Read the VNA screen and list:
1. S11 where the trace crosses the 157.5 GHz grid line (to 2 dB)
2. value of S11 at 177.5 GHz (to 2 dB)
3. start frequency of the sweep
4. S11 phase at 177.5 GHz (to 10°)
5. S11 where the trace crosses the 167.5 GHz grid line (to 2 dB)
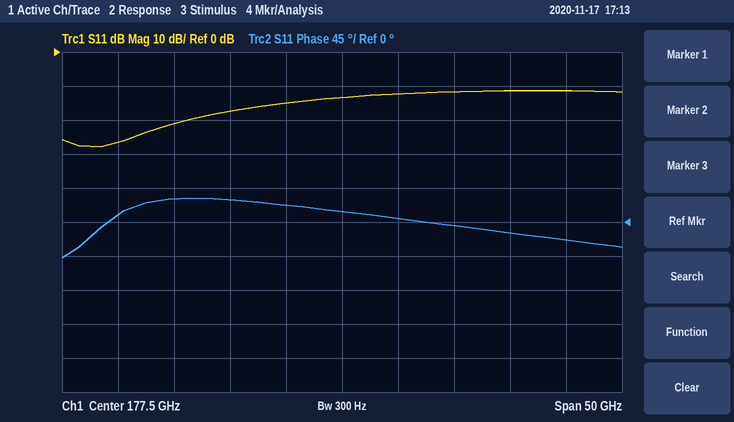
-26 dB
-14 dB
152.5 GHz
10°
-18 dB
